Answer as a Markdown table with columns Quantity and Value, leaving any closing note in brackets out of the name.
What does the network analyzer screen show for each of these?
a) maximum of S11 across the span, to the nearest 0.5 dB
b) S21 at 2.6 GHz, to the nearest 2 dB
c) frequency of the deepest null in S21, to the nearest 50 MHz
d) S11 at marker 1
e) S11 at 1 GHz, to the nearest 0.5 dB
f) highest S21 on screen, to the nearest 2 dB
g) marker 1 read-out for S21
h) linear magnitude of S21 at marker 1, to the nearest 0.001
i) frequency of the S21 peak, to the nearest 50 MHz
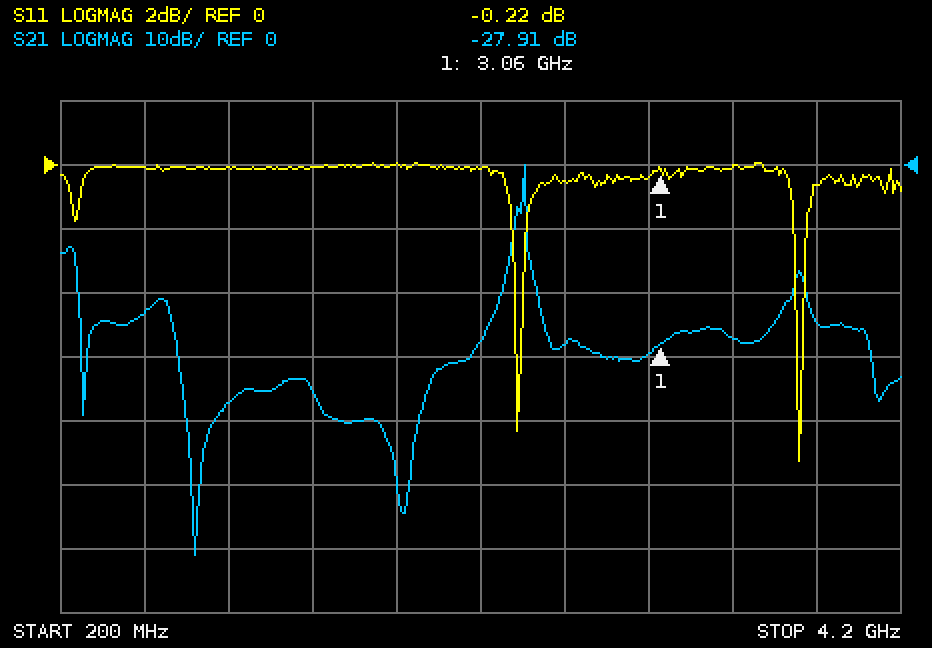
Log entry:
| Quantity | Value |
|---|---|
| maximum of S11 across the span, to the nearest 0.5 dB | 0.0 dB |
| S21 at 2.6 GHz, to the nearest 2 dB | -28 dB |
| frequency of the deepest null in S21, to the nearest 50 MHz | 850 MHz |
| S11 at marker 1 | -0.22 dB |
| S11 at 1 GHz, to the nearest 0.5 dB | 0.0 dB |
| highest S21 on screen, to the nearest 2 dB | 0 dB |
| marker 1 read-out for S21 | -27.91 dB |
| linear magnitude of S21 at marker 1, to the nearest 0.001 | 0.040 |
| frequency of the S21 peak, to the nearest 50 MHz | 2.40 GHz |
